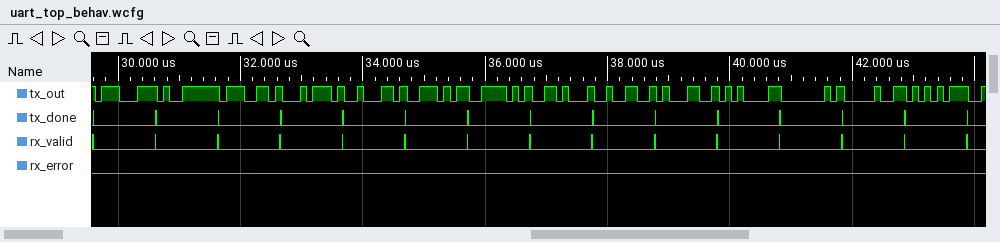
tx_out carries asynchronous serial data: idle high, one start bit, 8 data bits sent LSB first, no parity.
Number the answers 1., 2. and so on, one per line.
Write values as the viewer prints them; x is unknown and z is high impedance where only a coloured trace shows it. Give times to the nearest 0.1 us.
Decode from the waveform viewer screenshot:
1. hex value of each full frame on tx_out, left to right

1. C7, F9, 67, 74, 62, AE, 5E, 16, 32, 31, 85, 40, 90, D5
